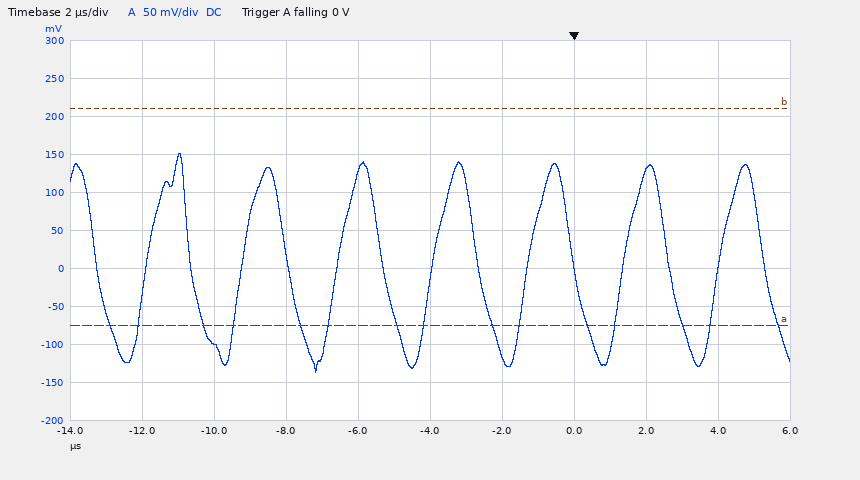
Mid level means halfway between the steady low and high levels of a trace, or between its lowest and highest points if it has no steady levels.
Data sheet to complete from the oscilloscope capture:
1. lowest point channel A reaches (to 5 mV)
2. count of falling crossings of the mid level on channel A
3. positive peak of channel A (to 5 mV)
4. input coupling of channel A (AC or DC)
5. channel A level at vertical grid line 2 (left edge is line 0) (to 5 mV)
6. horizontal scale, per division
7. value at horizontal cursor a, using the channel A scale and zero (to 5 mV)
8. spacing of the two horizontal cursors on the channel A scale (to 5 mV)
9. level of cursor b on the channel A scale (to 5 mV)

-135 mV
8
150 mV
DC
-100 mV
2 µs
-75 mV
285 mV
210 mV
